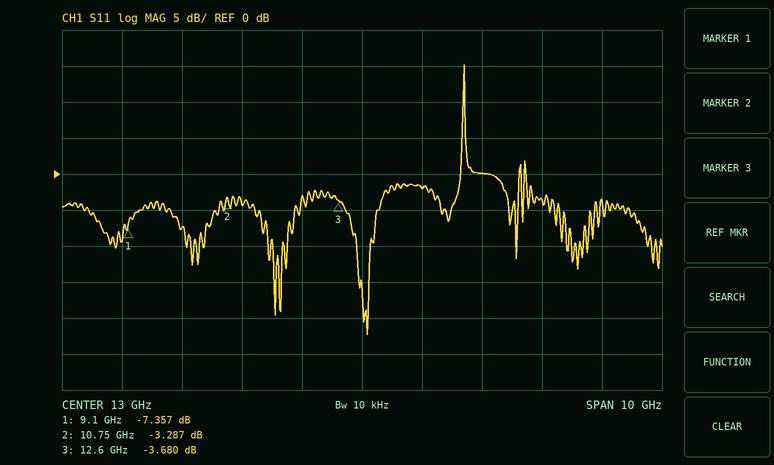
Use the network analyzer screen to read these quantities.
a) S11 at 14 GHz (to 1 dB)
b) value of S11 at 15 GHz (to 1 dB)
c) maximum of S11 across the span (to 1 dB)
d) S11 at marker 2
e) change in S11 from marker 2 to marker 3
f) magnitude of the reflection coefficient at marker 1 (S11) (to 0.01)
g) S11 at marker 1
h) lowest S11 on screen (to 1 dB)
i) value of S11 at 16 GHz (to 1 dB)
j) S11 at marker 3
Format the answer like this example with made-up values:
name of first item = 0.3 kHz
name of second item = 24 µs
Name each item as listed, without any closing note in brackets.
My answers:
S11 at 14 GHz = -2 dB
value of S11 at 15 GHz = 0 dB
maximum of S11 across the span = 15 dB
S11 at marker 2 = -3.287 dB
change in S11 from marker 2 to marker 3 = -0.393 dB
magnitude of the reflection coefficient at marker 1 (S11) = 0.43
S11 at marker 1 = -7.357 dB
lowest S11 on screen = -22 dB
value of S11 at 16 GHz = -4 dB
S11 at marker 3 = -3.680 dB
